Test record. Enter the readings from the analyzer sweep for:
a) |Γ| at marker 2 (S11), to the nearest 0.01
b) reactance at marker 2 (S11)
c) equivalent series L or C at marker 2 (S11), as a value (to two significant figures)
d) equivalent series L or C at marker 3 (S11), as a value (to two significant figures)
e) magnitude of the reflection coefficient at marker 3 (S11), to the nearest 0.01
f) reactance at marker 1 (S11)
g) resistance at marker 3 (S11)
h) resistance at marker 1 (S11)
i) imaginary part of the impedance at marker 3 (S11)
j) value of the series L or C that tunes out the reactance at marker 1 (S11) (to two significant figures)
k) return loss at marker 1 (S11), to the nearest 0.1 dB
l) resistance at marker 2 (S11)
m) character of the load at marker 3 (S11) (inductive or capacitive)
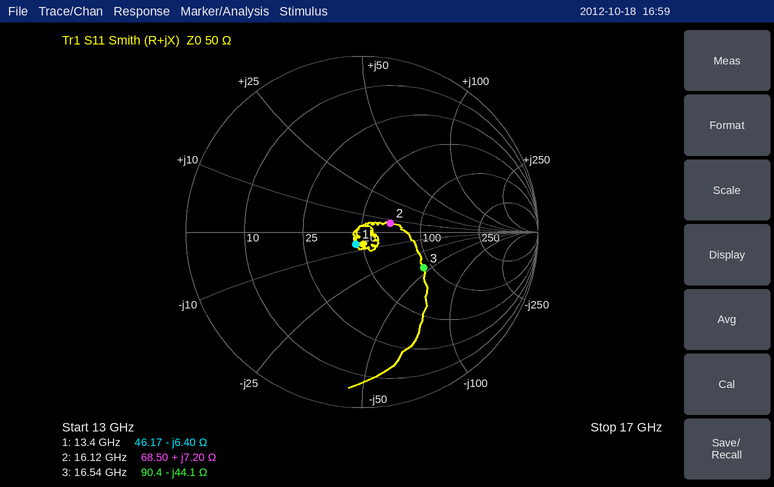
0.17
+7.20 Ω
71 pH
220 fF
0.41
-6.40 Ω
90.4 Ω
46.17 Ω
-44.1 Ω
76 pH
22.2 dB
68.50 Ω
capacitive
